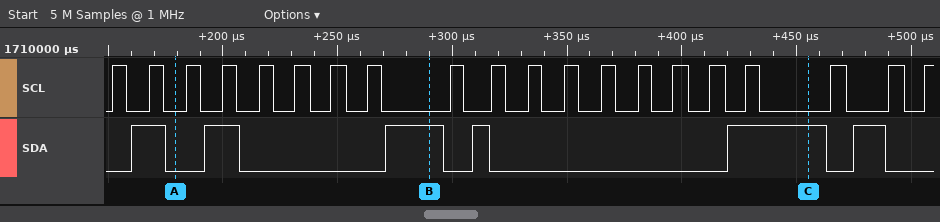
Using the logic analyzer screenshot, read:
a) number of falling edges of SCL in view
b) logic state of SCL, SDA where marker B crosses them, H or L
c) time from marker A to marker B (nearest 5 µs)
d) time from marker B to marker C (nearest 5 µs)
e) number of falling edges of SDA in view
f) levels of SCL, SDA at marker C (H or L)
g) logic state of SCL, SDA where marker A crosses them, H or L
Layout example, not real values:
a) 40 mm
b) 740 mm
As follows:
a) 19
b) SCL=L, SDA=H
c) 110 µs
d) 165 µs
e) 6
f) SCL=L, SDA=H
g) SCL=L, SDA=L
